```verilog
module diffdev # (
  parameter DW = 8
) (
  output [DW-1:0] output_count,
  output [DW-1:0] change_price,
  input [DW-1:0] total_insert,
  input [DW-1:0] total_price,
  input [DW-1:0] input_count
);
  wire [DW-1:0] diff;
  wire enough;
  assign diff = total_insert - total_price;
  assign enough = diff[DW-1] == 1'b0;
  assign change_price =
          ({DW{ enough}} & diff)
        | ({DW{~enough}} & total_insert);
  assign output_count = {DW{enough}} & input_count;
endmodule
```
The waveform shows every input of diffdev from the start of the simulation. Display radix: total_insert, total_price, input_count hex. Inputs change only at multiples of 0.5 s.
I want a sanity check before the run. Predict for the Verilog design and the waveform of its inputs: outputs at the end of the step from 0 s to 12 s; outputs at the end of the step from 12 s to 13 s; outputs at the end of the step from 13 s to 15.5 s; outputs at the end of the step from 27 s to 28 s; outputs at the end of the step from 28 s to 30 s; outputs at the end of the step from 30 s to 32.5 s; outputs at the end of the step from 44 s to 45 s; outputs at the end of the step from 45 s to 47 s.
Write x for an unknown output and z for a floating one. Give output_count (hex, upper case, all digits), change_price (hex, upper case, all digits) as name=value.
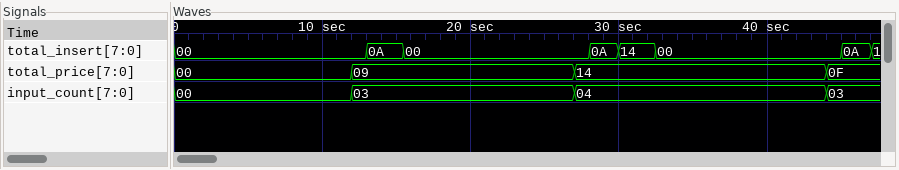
output_count=00, change_price=00
output_count=00, change_price=00
output_count=03, change_price=01
output_count=00, change_price=00
output_count=00, change_price=0A
output_count=04, change_price=00
output_count=00, change_price=00
output_count=00, change_price=0A
